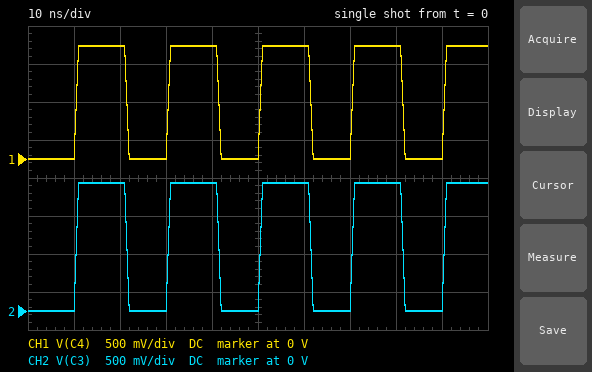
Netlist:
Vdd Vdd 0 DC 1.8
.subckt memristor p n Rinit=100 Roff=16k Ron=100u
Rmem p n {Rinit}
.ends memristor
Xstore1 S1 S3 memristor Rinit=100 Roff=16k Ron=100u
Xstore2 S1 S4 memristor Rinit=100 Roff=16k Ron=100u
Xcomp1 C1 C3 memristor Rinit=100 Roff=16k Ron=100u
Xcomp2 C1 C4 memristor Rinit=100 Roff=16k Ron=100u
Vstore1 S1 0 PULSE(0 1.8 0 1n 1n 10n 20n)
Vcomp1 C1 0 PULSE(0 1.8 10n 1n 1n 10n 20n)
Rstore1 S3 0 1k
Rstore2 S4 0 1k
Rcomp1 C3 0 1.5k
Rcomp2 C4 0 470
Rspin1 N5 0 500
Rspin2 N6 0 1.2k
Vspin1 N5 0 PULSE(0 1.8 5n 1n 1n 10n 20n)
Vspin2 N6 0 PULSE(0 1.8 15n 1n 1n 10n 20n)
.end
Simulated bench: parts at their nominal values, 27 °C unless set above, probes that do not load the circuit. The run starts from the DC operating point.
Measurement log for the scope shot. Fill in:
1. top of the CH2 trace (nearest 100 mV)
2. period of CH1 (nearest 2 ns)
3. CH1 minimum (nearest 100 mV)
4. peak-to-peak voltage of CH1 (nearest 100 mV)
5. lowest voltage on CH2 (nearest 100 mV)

1.7 V
20 ns
0 V
1.5 V
0 V
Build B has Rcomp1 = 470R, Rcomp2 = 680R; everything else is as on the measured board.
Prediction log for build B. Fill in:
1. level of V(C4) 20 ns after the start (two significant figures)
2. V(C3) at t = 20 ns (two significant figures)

1.6 V
1.5 V
